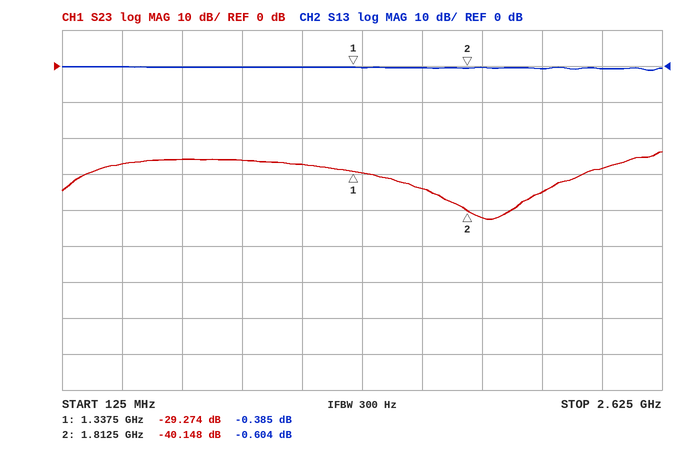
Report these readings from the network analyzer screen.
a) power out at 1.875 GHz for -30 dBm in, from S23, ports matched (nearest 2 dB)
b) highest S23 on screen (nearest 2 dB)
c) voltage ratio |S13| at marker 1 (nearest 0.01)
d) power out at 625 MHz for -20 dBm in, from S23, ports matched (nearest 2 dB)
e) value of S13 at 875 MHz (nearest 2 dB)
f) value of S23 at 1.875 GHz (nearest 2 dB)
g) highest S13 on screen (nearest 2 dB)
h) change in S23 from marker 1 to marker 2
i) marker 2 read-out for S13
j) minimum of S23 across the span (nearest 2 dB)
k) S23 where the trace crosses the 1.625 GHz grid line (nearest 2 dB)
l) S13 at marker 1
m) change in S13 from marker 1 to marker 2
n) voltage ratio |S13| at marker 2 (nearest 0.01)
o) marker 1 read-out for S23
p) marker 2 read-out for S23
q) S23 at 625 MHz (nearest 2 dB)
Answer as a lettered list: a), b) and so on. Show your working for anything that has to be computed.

a) -30 dBm + (-42 dB) = -72 dBm
b) -24 dB
c) 10^(-0.385/20) ≈ 0.96
d) -20 dBm + (-26 dB) = -46 dBm
e) 0 dB
f) -42 dB
g) 0 dB
h) -40.148 − (-29.274) = -10.874 dB
i) -0.604 dB
j) -42 dB
k) -34 dB
l) -0.385 dB
m) -0.604 − (-0.385) = -0.219 dB
n) 10^(-0.604/20) ≈ 0.93
o) -29.274 dB
p) -40.148 dB
q) -26 dB
